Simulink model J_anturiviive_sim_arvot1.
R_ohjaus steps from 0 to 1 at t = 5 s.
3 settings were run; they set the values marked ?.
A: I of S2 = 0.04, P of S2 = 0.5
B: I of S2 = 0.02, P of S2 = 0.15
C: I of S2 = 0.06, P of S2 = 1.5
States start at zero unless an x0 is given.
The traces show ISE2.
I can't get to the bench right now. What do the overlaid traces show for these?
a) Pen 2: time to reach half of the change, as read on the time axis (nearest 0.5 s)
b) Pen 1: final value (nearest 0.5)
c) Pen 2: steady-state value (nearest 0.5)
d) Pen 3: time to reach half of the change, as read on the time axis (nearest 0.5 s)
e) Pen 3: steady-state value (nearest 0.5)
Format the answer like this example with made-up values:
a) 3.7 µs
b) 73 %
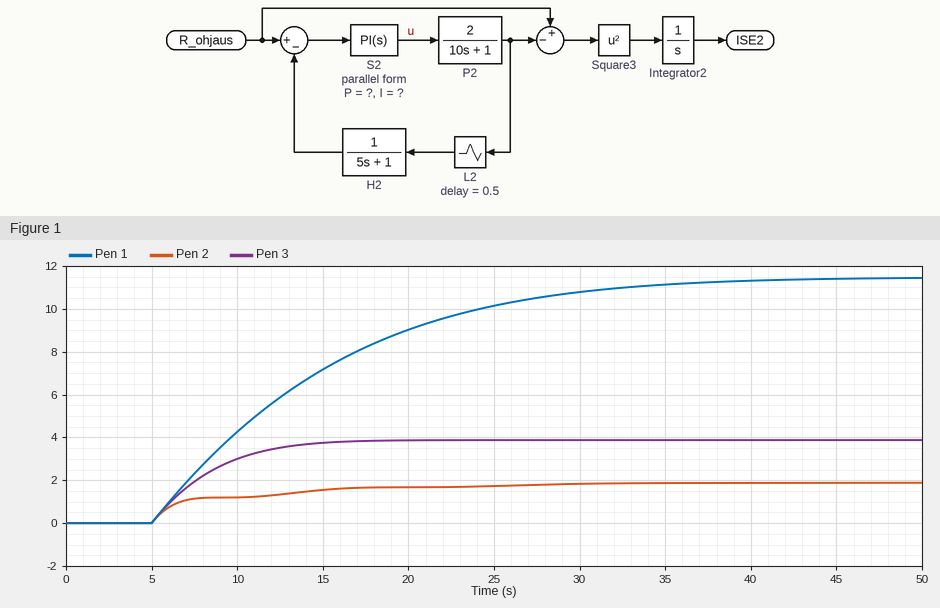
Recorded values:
a) 6.5 s
b) 11.5
c) 2.0
d) 7.5 s
e) 4.0
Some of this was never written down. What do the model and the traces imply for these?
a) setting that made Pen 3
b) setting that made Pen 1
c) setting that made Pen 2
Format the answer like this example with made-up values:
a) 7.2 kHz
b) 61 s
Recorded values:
a) A
b) B
c) C
